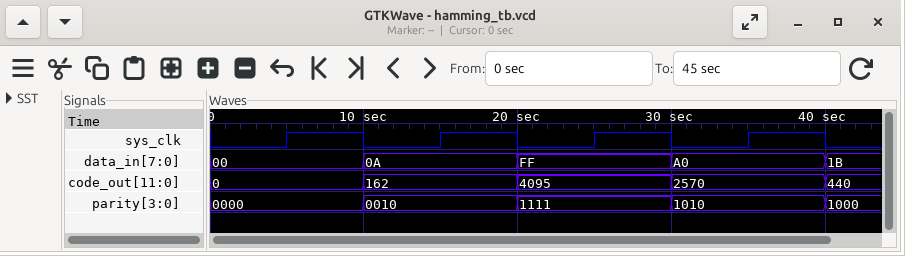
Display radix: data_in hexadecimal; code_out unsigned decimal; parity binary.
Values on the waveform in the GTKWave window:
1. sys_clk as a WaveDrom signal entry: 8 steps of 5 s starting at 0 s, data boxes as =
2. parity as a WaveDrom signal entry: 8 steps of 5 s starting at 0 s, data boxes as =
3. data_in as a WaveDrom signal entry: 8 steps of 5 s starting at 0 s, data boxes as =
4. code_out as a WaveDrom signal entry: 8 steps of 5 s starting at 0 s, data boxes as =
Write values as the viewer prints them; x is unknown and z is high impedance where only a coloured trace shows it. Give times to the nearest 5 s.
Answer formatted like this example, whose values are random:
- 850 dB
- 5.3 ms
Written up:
- {name: 'sys_clk', wave: '01010101'}
- {name: 'parity', wave: '=.=.=.=.', data: '0000 0010 1111 1010'}
- {name: 'data_in', wave: '=.=.=.=.', data: '00 0A FF A0'}
- {name: 'code_out', wave: '=.=.=.=.', data: '0 162 4095 2570'}
